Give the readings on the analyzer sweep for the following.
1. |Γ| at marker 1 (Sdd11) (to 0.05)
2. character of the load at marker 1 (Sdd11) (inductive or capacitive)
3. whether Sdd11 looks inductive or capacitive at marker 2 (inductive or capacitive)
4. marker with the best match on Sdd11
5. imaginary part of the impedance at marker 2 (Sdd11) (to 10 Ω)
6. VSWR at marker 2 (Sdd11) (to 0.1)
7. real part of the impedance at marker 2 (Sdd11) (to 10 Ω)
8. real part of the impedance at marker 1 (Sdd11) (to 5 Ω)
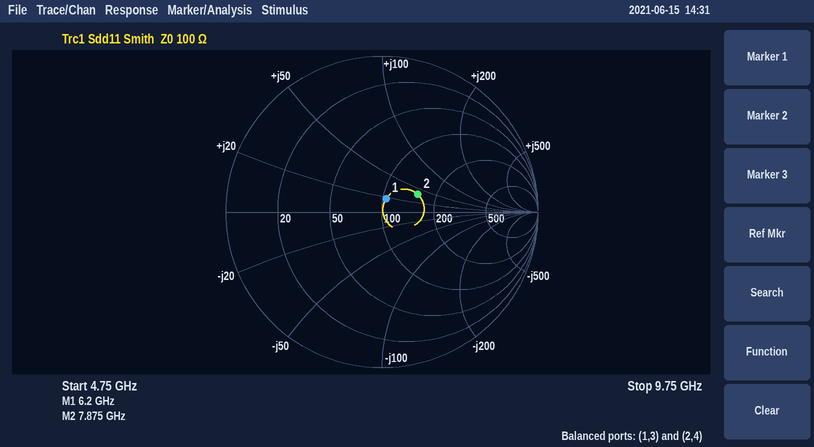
0.10
inductive
inductive
marker 1
+40 Ω
1.7
150 Ω
105 Ω
